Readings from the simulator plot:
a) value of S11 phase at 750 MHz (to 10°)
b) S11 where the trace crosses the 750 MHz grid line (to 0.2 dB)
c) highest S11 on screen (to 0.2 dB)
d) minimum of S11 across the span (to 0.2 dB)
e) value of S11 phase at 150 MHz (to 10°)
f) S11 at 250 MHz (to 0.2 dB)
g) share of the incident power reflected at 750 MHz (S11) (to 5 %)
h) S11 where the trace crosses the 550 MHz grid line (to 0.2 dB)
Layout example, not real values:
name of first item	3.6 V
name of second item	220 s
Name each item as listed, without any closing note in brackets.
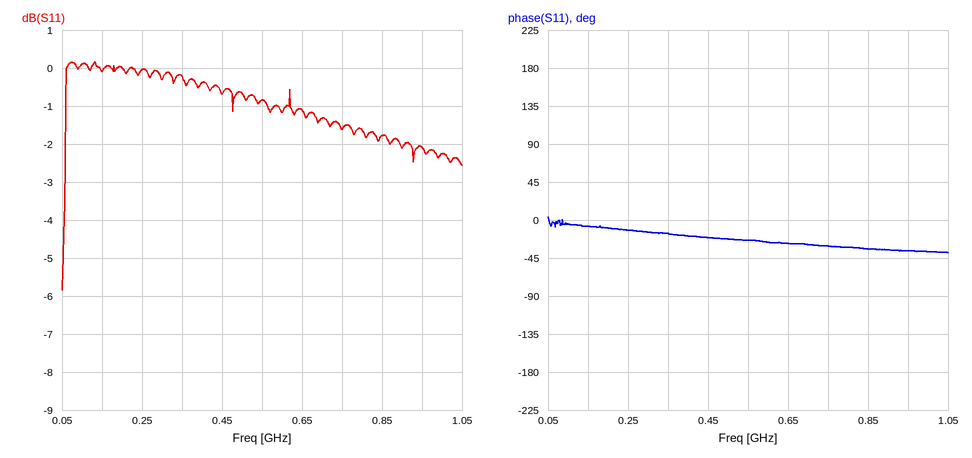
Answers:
value of S11 phase at 750 MHz	-30°
S11 where the trace crosses the 750 MHz grid line	-1.6 dB
highest S11 on screen	0.2 dB
minimum of S11 across the span	-5.8 dB
value of S11 phase at 150 MHz	-10°
S11 at 250 MHz	0.0 dB
share of the incident power reflected at 750 MHz (S11)	70 %
S11 where the trace crosses the 550 MHz grid line	-0.8 dB
